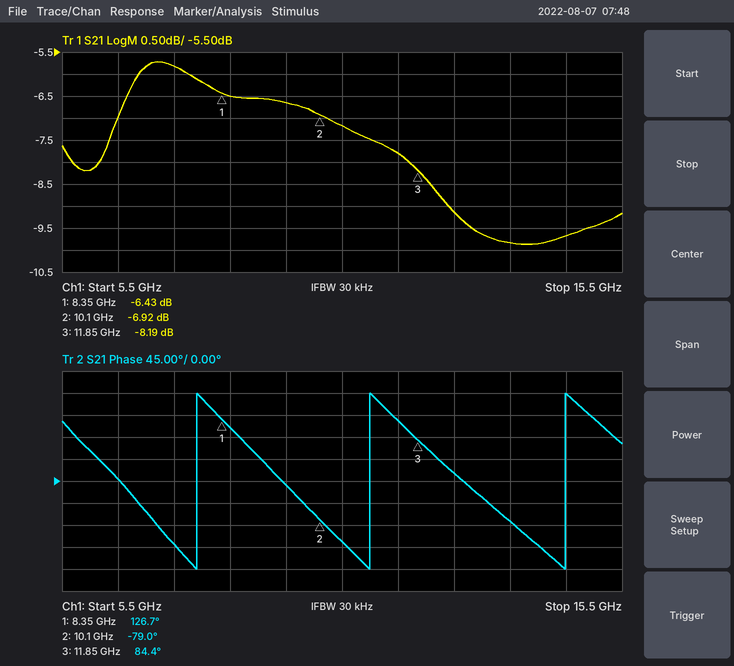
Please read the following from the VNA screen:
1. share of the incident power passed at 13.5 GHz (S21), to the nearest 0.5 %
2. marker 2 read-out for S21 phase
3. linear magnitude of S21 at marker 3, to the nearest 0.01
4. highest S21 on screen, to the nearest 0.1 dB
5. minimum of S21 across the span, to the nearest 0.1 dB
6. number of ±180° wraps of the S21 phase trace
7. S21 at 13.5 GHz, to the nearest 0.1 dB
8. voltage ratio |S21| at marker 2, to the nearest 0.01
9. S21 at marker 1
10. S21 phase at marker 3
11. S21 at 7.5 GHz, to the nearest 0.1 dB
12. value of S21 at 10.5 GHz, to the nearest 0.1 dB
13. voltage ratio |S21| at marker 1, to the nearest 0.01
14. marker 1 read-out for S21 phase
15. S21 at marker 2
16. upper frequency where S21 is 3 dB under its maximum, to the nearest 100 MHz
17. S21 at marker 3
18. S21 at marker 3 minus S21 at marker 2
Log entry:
10.5 %
-79.0°
0.39
-5.7 dB
-9.9 dB
3
-9.8 dB
0.45
-6.43 dB
84.4°
-5.8 dB
-7.2 dB
0.48
126.7°
-6.92 dB
12.2 GHz
-8.19 dB
-1.27 dB
